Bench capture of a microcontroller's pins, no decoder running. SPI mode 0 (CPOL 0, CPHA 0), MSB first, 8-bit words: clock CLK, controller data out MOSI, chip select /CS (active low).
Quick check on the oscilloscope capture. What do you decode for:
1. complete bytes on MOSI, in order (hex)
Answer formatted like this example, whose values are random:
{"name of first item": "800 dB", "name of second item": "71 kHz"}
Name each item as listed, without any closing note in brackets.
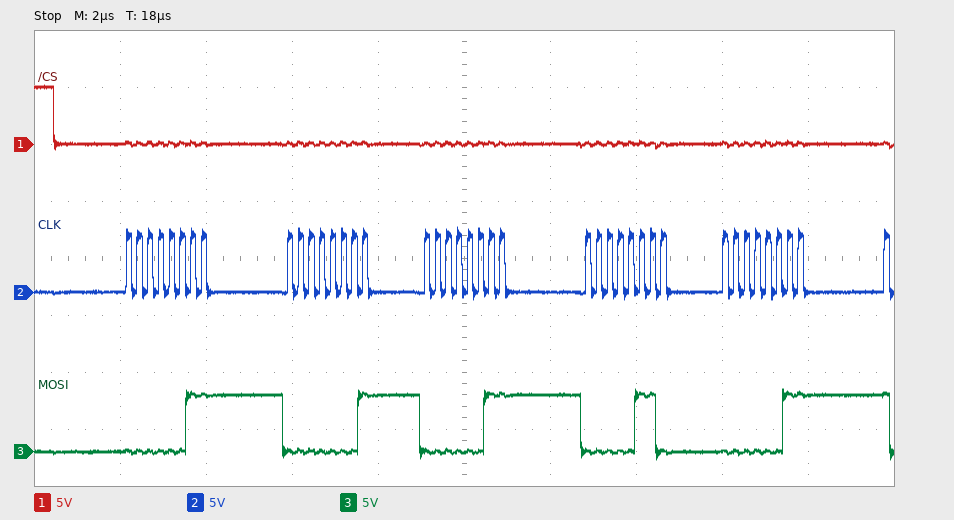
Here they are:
{"complete bytes on MOSI, in order": "03 01 03 06 03"}
